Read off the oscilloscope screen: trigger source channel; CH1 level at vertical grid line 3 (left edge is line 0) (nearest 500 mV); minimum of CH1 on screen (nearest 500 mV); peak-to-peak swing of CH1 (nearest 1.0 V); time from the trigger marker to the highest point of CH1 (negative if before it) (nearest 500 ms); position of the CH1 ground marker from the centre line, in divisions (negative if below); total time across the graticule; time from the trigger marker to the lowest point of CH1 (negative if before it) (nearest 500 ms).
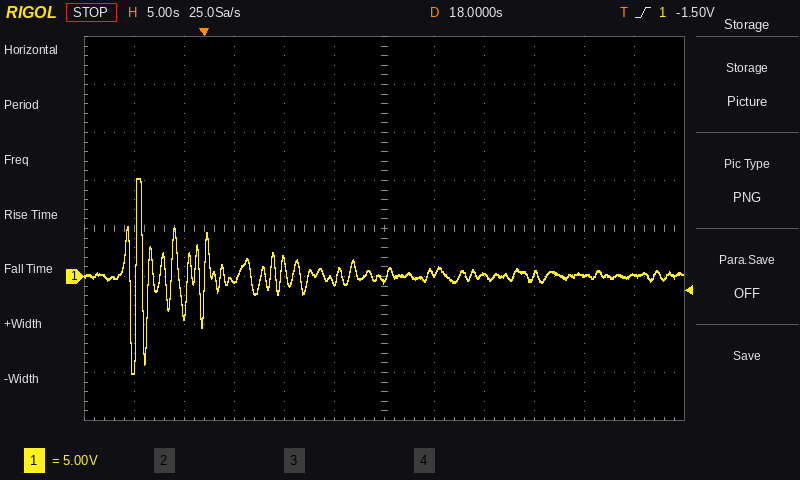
CH1
-500 mV
-10.0 V
20.0 V
-6.5 s
-1.0 div
60 s
-7.0 s
